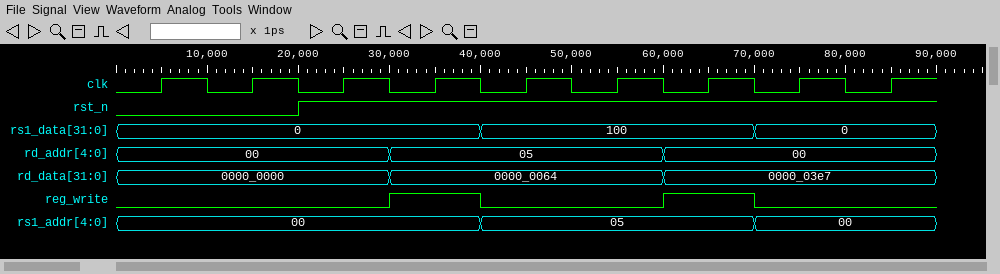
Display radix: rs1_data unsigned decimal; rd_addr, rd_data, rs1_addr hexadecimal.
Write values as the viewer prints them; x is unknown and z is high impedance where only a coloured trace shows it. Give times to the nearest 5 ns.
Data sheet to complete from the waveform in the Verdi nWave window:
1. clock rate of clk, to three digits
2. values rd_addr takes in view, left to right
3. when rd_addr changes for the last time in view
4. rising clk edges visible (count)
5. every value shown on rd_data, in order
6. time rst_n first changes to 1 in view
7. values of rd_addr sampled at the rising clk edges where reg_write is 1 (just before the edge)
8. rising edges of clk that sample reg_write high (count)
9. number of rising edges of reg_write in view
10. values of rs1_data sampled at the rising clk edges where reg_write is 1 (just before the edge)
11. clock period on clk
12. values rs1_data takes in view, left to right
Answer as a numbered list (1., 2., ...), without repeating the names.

1. 100 MHz
2. 00, 05, 00
3. 60 ns
4. 9
5. 0000_0000, 0000_0064, 0000_03e7
6. 20 ns
7. 05, 00
8. 2
9. 2
10. 0, 100
11. 10 ns
12. 0, 100, 0
